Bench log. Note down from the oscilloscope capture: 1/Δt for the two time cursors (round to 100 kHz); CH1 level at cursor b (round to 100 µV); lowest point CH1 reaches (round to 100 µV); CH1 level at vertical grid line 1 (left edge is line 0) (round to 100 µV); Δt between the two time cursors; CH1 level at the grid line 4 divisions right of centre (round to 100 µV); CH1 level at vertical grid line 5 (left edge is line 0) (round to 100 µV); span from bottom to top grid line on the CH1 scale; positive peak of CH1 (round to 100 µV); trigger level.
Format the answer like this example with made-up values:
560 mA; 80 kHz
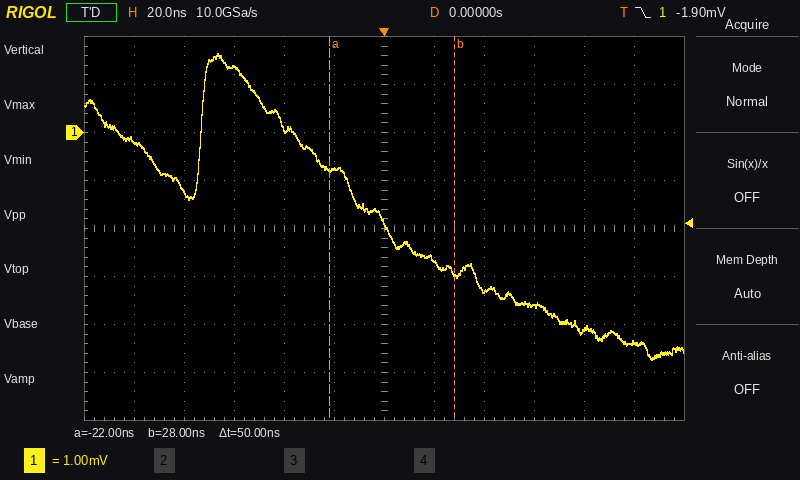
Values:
20.0 MHz; -2.9 mV; -4.7 mV; -200 µV; 50 ns; -4.1 mV; -800 µV; 8 mV; 1.6 mV; -1.90 mV
